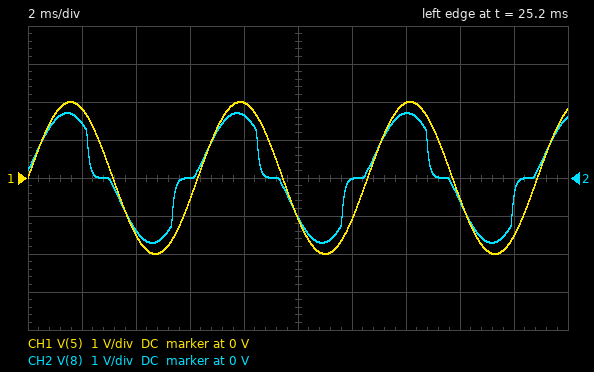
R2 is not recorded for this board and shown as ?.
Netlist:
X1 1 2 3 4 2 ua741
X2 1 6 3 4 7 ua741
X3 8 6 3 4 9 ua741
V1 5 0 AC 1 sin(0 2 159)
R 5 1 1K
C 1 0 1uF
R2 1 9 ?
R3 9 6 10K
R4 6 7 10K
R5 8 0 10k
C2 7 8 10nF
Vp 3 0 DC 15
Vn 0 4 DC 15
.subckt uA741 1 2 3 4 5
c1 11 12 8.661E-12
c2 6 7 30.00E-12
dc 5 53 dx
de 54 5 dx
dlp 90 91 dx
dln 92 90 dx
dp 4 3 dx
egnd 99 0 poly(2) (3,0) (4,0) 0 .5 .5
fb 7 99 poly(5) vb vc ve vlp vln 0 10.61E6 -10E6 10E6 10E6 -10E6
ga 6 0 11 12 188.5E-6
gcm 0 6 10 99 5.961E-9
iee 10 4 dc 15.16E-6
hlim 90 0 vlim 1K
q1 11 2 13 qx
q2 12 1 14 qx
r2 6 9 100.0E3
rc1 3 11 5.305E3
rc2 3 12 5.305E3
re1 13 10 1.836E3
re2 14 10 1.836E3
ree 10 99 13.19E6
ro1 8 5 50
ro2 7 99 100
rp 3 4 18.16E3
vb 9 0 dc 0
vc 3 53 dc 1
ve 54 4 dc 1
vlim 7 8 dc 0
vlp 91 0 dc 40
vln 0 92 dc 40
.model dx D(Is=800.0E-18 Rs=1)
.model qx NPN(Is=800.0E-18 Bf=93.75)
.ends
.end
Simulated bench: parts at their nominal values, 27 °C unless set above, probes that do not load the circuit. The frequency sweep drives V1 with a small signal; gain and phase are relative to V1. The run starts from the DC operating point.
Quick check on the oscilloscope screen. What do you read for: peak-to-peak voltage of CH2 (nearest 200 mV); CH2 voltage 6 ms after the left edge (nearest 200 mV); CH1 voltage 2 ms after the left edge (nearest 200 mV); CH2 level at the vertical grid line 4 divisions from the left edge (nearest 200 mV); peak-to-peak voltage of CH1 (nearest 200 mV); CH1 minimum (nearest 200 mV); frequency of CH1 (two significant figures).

3.4 V
0 V
1.8 V
1.6 V
4.0 V
-2.0 V
160 Hz
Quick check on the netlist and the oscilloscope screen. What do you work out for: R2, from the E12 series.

8.2 kΩ
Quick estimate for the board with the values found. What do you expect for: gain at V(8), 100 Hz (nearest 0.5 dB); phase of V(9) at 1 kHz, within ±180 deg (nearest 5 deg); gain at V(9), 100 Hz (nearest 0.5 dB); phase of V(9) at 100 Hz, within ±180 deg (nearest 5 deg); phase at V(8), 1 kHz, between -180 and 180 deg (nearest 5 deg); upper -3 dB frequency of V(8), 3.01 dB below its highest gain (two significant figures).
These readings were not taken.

-4.5 dB
-25 deg
19.5 dB
140 deg
-80 deg
270 Hz
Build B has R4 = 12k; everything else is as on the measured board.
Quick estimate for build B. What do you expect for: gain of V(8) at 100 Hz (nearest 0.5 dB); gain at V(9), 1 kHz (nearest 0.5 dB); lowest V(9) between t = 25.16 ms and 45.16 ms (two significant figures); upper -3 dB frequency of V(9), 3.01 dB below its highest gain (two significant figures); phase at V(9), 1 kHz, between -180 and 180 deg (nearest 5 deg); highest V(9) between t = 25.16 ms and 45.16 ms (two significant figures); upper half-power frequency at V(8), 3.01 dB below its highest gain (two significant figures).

-3.0 dB
-11.5 dB
-12 V
190 Hz
-30 deg
12 V
260 Hz
